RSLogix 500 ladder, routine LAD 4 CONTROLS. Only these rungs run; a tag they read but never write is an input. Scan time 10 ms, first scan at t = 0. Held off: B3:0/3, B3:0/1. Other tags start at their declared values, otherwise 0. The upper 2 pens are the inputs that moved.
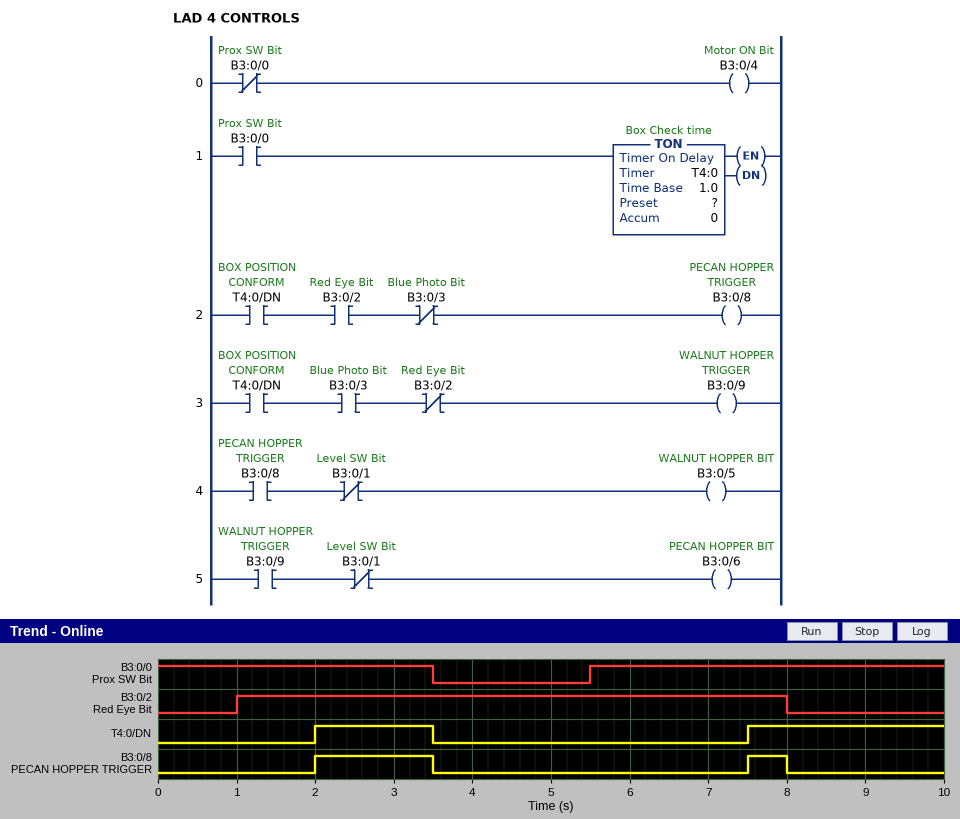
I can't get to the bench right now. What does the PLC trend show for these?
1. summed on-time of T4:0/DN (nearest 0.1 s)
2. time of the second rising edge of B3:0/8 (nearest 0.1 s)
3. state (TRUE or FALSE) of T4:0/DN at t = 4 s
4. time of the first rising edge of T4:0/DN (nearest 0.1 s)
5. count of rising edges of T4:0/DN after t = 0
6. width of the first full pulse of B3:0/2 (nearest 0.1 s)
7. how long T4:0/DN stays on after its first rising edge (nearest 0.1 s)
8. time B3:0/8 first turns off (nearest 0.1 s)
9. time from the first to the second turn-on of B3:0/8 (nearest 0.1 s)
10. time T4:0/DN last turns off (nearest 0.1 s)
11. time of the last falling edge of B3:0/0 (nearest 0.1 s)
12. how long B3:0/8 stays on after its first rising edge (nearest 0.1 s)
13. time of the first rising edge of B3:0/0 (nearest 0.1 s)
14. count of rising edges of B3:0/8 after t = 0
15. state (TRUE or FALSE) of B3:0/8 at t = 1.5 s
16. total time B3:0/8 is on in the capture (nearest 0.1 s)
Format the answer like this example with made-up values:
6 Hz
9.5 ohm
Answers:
4.0 s
7.5 s
FALSE
2.0 s
2
7.0 s
1.5 s
3.5 s
5.5 s
3.5 s
3.5 s
1.5 s
5.5 s
2
FALSE
2.0 s
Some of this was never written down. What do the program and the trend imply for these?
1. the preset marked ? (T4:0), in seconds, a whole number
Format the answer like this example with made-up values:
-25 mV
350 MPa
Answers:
2 s
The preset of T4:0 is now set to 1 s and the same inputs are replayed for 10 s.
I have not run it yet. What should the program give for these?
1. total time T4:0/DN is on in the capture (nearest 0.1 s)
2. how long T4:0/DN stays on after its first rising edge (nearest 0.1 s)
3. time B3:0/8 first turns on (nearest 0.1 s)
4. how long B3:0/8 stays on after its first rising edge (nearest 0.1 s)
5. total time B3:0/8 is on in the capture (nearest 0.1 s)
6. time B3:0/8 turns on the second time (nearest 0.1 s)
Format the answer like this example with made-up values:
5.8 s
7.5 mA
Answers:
6.0 s
2.5 s
1.0 s
2.5 s
4.0 s
6.5 s
